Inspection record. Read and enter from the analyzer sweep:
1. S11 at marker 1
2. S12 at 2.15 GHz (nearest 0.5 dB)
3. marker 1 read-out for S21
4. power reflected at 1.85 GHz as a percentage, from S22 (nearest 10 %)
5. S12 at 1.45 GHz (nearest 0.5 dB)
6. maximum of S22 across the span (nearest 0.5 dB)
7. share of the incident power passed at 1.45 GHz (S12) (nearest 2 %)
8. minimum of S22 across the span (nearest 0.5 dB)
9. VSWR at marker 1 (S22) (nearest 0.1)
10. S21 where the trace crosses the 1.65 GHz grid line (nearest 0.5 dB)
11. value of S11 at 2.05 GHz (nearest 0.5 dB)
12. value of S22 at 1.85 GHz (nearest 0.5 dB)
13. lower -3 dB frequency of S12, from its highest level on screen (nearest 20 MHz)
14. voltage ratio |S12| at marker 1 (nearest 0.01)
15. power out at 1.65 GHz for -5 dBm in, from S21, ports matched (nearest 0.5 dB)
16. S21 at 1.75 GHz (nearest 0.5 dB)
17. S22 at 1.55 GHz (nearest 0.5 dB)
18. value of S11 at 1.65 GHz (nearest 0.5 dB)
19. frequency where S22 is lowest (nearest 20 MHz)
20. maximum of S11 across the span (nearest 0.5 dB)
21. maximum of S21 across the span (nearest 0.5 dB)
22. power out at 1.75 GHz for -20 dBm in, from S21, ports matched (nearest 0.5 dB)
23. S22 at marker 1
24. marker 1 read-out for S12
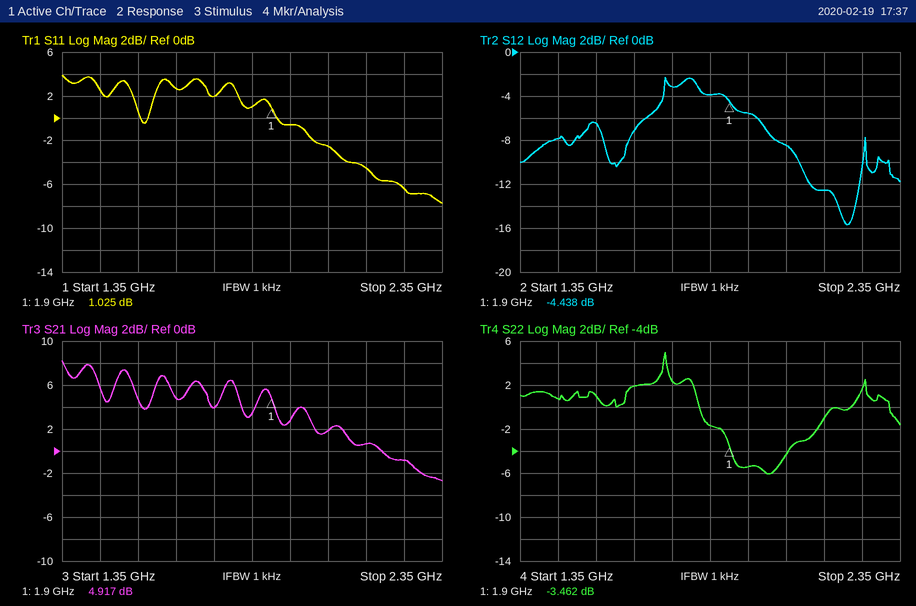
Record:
1.025 dB
-12.5 dB
4.917 dB
70 %
-8.0 dB
5.0 dB
16 %
-6.0 dB
5.1
5.0 dB
-2.5 dB
-1.5 dB
1.70 GHz
0.60
0.0 dBm
4.0 dB
1.0 dB
2.5 dB
2.00 GHz
4.0 dB
8.0 dB
-16.0 dBm
-3.462 dB
-4.438 dB
